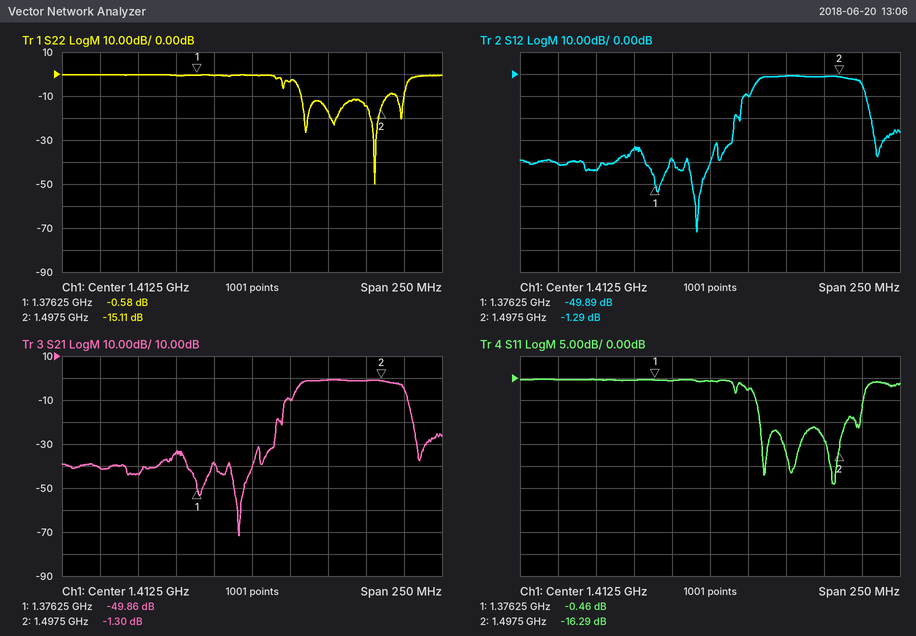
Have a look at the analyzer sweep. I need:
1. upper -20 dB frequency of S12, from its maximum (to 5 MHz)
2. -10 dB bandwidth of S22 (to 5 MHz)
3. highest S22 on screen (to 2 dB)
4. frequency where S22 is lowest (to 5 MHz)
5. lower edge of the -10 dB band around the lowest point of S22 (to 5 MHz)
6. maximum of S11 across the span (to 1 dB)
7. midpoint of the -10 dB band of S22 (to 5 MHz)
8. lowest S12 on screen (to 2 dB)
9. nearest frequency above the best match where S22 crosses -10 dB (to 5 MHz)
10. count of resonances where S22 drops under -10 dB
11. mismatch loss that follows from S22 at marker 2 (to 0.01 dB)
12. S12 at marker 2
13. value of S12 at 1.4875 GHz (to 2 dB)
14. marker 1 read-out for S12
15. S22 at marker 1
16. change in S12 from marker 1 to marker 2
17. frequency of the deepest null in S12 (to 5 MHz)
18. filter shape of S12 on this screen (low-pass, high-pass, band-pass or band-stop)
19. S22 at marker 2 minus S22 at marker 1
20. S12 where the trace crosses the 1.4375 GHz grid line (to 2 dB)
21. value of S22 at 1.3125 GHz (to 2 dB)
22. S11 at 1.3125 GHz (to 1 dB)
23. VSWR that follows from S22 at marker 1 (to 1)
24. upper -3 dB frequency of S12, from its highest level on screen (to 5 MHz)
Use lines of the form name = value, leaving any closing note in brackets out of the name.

upper -20 dB frequency of S12, from its maximum = 1.520 GHz
-10 dB bandwidth of S22 = 55 MHz
highest S22 on screen = 0 dB
frequency where S22 is lowest = 1.495 GHz
lower edge of the -10 dB band around the lowest point of S22 = 1.445 GHz
maximum of S11 across the span = 0 dB
midpoint of the -10 dB band of S22 = 1.475 GHz
lowest S12 on screen = -72 dB
nearest frequency above the best match where S22 crosses -10 dB = 1.500 GHz
count of resonances where S22 drops under -10 dB = 4
mismatch loss that follows from S22 at marker 2 = 0.14 dB
S12 at marker 2 = -1.29 dB
value of S12 at 1.4875 GHz = -2 dB
marker 1 read-out for S12 = -49.89 dB
S22 at marker 1 = -0.58 dB
change in S12 from marker 1 to marker 2 = 48.60 dB
frequency of the deepest null in S12 = 1.405 GHz
filter shape of S12 on this screen = band-pass
S22 at marker 2 minus S22 at marker 1 = -14.53 dB
S12 where the trace crosses the 1.4375 GHz grid line = -10 dB
value of S22 at 1.3125 GHz = 0 dB
S11 at 1.3125 GHz = 0 dB
VSWR that follows from S22 at marker 1 = 30
upper -3 dB frequency of S12, from its highest level on screen = 1.510 GHz
